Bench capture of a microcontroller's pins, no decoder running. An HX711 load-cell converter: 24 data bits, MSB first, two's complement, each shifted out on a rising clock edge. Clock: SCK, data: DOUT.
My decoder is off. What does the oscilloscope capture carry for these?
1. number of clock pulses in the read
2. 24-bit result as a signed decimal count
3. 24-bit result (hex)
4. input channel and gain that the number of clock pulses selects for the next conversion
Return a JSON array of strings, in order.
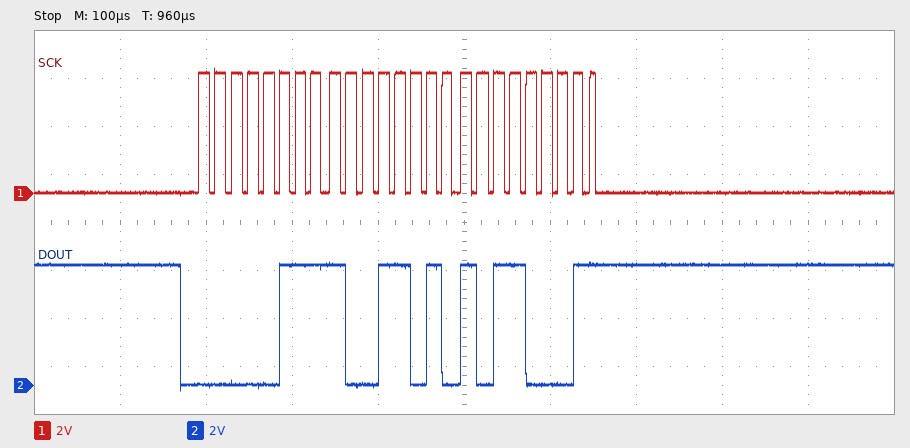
["25", "498353", "0x079AB1", "channel A, gain 128"]
